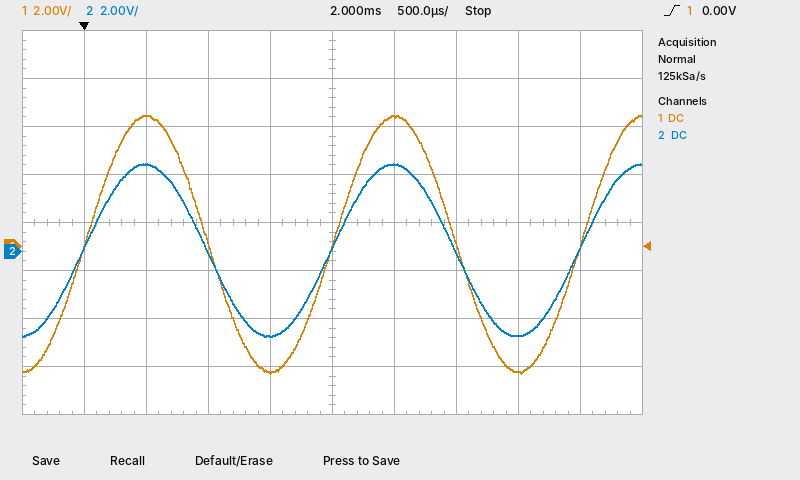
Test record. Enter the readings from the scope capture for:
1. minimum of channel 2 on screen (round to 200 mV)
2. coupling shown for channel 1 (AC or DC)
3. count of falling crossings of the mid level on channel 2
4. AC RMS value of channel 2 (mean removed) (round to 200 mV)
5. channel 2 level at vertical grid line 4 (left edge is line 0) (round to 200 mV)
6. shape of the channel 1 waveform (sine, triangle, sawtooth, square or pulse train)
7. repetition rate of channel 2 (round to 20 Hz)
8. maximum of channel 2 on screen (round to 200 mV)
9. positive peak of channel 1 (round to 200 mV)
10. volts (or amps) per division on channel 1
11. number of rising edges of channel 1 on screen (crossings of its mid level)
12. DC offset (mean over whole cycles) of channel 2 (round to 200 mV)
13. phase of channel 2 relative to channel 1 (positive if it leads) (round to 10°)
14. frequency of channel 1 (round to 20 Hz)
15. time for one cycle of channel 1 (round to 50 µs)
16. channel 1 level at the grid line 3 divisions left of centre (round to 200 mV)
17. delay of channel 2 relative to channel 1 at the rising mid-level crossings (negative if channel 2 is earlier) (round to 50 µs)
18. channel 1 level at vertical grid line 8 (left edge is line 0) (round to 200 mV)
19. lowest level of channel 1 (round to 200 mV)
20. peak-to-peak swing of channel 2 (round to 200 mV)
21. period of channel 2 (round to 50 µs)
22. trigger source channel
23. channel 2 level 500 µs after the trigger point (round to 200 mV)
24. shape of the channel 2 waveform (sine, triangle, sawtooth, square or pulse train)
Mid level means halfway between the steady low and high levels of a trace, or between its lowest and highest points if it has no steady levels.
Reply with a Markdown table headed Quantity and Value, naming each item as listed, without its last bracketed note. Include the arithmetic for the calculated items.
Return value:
| Quantity | Value |
|---|---|
| minimum of channel 2 on screen | -3.6 V |
| coupling shown for channel 1 | DC |
| count of falling crossings of the mid level on channel 2 | 2 |
| AC RMS value of channel 2 (mean removed) | 7.2 V / (2√2) ≈ 2.6 V |
| channel 2 level at vertical grid line 4 (left edge is line 0) | -3.6 V |
| shape of the channel 1 waveform | sine |
| repetition rate of channel 2 | 1 / 2.00 ms ≈ 500 Hz |
| maximum of channel 2 on screen | 3.6 V |
| positive peak of channel 1 | 5.4 V |
| volts (or amps) per division on channel 1 | 2 V |
| number of rising edges of channel 1 on screen | 3 |
| DC offset (mean over whole cycles) of channel 2 | (3.6 V + (-3.6 V)) / 2 ≈ 0.0 V |
| phase of channel 2 relative to channel 1 (positive if it leads) | −360° × (0 µs) / 2.00 ms ≈ 0° |
| frequency of channel 1 | 1 / 2.00 ms ≈ 500 Hz |
| time for one cycle of channel 1 | 2.00 ms |
| channel 1 level at the grid line 3 divisions left of centre | 5.4 V |
| delay of channel 2 relative to channel 1 at the rising mid-level crossings (negative if channel 2 is earlier) | 0 µs |
| channel 1 level at vertical grid line 8 (left edge is line 0) | -5.2 V |
| lowest level of channel 1 | -5.2 V |
| peak-to-peak swing of channel 2 | 3.6 V − (-3.6 V) = 7.2 V |
| period of channel 2 | 2.00 ms |
| trigger source channel | channel 1 |
| channel 2 level 500 µs after the trigger point | 3.6 V |
| shape of the channel 2 waveform | sine |
